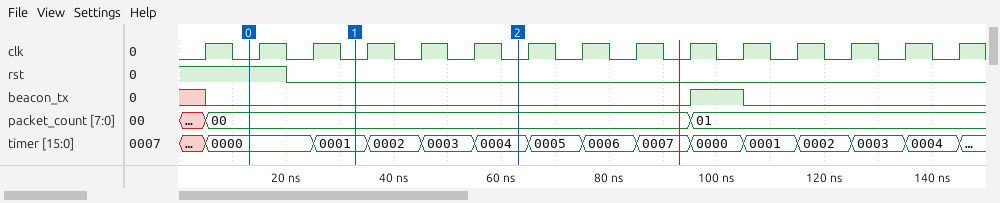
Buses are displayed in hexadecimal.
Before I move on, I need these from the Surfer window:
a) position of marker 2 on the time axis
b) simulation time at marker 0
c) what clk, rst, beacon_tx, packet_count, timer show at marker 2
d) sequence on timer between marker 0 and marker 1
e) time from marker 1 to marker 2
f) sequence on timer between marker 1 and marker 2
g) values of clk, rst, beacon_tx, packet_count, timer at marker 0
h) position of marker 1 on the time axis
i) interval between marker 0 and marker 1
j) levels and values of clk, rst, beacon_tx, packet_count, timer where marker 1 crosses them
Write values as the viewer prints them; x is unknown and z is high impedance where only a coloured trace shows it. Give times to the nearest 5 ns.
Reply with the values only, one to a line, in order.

65 ns
15 ns
clk=0, rst=0, beacon_tx=0, packet_count=00, timer=0004
0000, 0001
30 ns
0001, 0002, 0003, 0004
clk=0, rst=1, beacon_tx=0, packet_count=00, timer=0000
35 ns
20 ns
clk=0, rst=0, beacon_tx=0, packet_count=00, timer=0001
